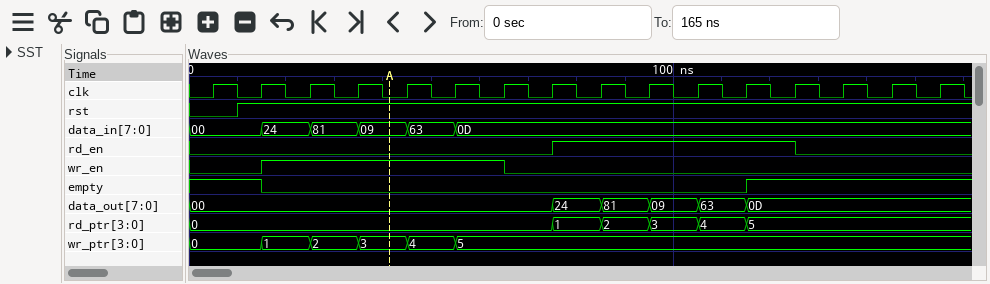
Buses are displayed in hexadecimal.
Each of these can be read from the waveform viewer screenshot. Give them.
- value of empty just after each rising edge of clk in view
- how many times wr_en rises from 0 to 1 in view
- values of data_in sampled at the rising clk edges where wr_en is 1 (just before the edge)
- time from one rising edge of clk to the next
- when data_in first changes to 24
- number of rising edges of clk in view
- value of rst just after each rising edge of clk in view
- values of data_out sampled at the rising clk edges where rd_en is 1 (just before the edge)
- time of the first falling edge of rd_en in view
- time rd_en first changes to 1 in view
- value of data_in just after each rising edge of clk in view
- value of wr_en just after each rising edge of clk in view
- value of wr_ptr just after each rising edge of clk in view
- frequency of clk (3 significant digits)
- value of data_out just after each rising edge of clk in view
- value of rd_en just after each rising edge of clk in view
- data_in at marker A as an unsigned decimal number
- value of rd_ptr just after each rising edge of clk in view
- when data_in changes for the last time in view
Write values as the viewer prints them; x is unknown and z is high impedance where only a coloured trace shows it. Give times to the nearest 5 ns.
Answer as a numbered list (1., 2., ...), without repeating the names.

1. 1 0 0 0 0 0 0 0 0 0 0 1 1 1 1 1
2. 1
3. 24, 81, 09, 63, 0D
4. 10 ns
5. 15 ns
6. 16
7. 0 1 1 1 1 1 1 1 1 1 1 1 1 1 1 1
8. 24, 81, 09, 63, 0D
9. 125 ns
10. 75 ns
11. 00, 24, 81, 09, 63, 0D, 0D, 0D, 0D, 0D, 0D, 0D, 0D, 0D, 0D, 0D
12. 0 1 1 1 1 1 0 0 0 0 0 0 0 0 0 0
13. 0, 1, 2, 3, 4, 5, 5, 5, 5, 5, 5, 5, 5, 5, 5, 5
14. 100 MHz
15. 00, 00, 00, 00, 00, 00, 00, 24, 81, 09, 63, 0D, 0D, 0D, 0D, 0D
16. 0 0 0 0 0 0 0 1 1 1 1 1 0 0 0 0
17. 9
18. 0, 0, 0, 0, 0, 0, 0, 1, 2, 3, 4, 5, 5, 5, 5, 5
19. 55 ns
